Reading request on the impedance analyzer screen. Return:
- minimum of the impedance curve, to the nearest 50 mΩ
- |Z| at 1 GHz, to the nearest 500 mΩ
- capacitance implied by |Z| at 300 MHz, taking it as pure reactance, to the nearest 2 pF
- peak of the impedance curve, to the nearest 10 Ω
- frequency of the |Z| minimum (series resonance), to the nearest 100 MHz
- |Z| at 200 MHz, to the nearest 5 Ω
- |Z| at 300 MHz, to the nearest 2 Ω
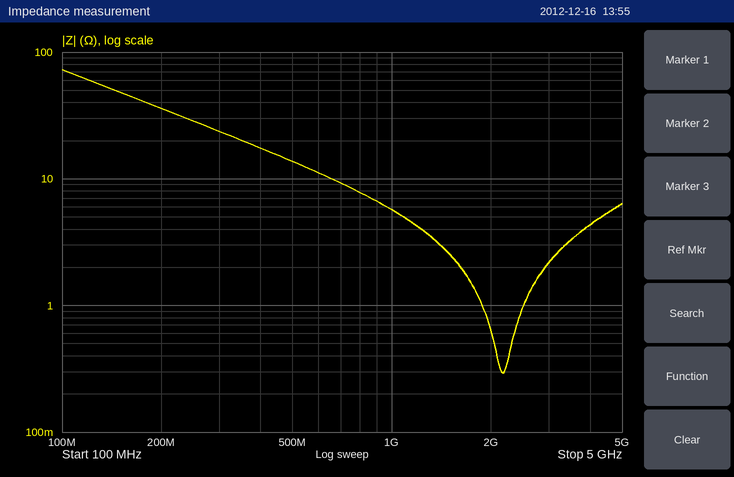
300 mΩ
5.5 Ω
22 pF
70 Ω
2.2 GHz
35 Ω
24 Ω
